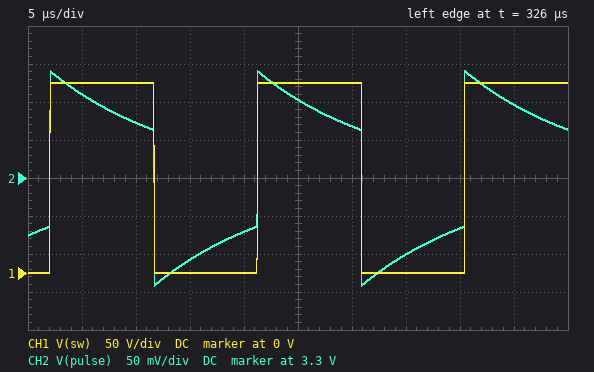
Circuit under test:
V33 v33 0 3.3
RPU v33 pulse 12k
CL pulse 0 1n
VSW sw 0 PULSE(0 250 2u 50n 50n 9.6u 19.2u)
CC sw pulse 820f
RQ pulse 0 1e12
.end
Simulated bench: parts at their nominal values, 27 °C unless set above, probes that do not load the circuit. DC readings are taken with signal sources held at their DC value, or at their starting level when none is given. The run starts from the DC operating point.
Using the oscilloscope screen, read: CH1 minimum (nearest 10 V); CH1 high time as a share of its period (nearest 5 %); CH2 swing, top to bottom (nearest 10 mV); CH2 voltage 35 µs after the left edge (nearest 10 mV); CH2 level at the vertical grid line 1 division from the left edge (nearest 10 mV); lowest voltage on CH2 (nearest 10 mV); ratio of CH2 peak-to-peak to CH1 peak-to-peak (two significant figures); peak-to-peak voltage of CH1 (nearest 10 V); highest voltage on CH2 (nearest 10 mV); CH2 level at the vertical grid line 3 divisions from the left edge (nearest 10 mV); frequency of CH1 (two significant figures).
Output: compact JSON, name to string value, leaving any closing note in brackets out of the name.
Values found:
{"CH1 minimum": "0 V", "CH1 high time as a share of its period": "50 %", "CH2 swing, top to bottom": "280 mV", "CH2 voltage 35 µs after the left edge": "3.20 V", "CH2 level at the vertical grid line 1 division from the left edge": "3.41 V", "lowest voltage on CH2": "3.16 V", "ratio of CH2 peak-to-peak to CH1 peak-to-peak": "0.0011", "peak-to-peak voltage of CH1": "250 V", "highest voltage on CH2": "3.44 V", "CH2 level at the vertical grid line 3 divisions from the left edge": "3.19 V", "frequency of CH1": "52 kHz"}
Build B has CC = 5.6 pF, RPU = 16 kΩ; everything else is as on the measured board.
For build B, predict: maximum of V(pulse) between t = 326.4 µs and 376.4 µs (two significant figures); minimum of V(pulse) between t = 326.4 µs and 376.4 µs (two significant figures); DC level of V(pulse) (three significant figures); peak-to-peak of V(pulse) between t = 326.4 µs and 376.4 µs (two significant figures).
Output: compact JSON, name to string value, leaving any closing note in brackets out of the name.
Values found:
{"maximum of V(pulse) between t = 326.4 µs and 376.4 µs": "4.2 V", "minimum of V(pulse) between t = 326.4 µs and 376.4 µs": "2.4 V", "DC level of V(pulse)": "3.30 V", "peak-to-peak of V(pulse) between t = 326.4 µs and 376.4 µs": "1.8 V"}
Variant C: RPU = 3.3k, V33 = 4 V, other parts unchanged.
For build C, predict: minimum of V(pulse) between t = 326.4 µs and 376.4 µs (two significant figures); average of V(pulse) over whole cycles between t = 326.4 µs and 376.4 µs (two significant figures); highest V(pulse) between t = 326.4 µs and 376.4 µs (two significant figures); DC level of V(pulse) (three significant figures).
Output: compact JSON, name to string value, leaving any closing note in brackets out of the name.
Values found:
{"minimum of V(pulse) between t = 326.4 µs and 376.4 µs": "3.8 V", "average of V(pulse) over whole cycles between t = 326.4 µs and 376.4 µs": "4.0 V", "highest V(pulse) between t = 326.4 µs and 376.4 µs": "4.2 V", "DC level of V(pulse)": "4.00 V"}
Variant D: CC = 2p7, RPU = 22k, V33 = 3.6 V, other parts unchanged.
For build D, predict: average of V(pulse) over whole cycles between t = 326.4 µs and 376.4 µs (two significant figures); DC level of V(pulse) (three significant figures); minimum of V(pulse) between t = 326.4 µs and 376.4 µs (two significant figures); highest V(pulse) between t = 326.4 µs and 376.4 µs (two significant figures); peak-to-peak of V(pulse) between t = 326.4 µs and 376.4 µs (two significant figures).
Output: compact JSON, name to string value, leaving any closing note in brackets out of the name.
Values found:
{"average of V(pulse) over whole cycles between t = 326.4 µs and 376.4 µs": "3.6 V", "DC level of V(pulse)": "3.60 V", "minimum of V(pulse) between t = 326.4 µs and 376.4 µs": "3.2 V", "highest V(pulse) between t = 326.4 µs and 376.4 µs": "4.0 V", "peak-to-peak of V(pulse) between t = 326.4 µs and 376.4 µs": "820 mV"}
